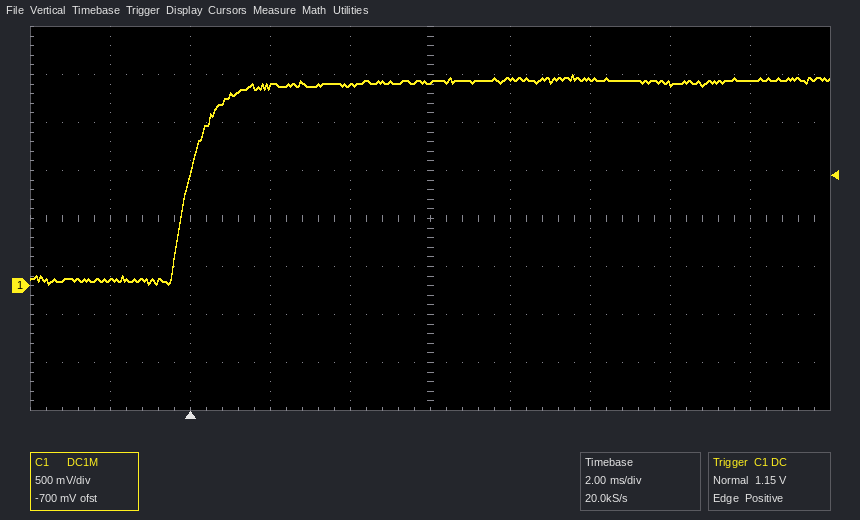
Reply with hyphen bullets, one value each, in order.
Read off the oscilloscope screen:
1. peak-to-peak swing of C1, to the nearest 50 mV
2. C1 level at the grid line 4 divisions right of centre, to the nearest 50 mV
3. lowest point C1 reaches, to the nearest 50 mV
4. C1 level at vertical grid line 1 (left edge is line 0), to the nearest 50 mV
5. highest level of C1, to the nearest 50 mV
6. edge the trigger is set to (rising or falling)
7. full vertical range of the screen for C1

- 2.20 V
- 2.15 V
- 0 mV
- 50 mV
- 2.20 V
- rising
- 4 V
